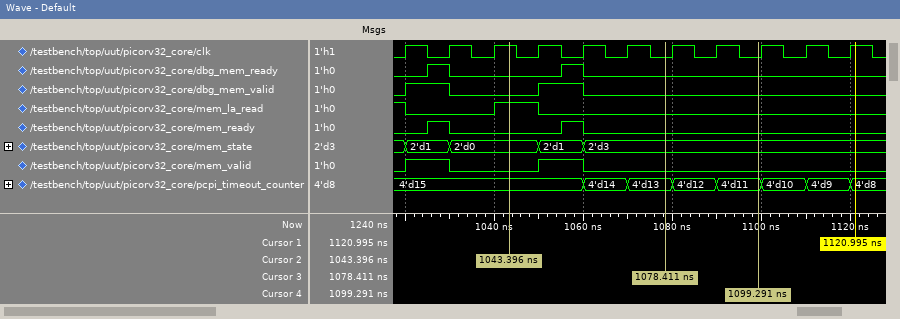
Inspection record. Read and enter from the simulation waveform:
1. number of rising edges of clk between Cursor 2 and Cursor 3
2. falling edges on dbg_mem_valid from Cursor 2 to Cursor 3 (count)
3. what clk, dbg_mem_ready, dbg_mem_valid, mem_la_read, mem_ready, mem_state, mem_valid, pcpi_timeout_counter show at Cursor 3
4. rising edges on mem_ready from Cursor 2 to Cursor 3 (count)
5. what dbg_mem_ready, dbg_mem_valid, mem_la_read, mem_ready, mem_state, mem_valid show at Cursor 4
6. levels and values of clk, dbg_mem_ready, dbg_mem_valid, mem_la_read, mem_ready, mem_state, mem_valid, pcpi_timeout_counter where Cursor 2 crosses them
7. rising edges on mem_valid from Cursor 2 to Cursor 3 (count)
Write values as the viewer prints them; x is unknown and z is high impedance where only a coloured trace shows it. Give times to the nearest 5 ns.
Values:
3
1
clk=0, dbg_mem_ready=0, dbg_mem_valid=0, mem_la_read=0, mem_ready=0, mem_state=2'd3, mem_valid=0, pcpi_timeout_counter=4'd13
1
dbg_mem_ready=0, dbg_mem_valid=0, mem_la_read=0, mem_ready=0, mem_state=2'd3, mem_valid=0
clk=1, dbg_mem_ready=0, dbg_mem_valid=0, mem_la_read=1, mem_ready=0, mem_state=2'd0, mem_valid=0, pcpi_timeout_counter=4'd15
1
